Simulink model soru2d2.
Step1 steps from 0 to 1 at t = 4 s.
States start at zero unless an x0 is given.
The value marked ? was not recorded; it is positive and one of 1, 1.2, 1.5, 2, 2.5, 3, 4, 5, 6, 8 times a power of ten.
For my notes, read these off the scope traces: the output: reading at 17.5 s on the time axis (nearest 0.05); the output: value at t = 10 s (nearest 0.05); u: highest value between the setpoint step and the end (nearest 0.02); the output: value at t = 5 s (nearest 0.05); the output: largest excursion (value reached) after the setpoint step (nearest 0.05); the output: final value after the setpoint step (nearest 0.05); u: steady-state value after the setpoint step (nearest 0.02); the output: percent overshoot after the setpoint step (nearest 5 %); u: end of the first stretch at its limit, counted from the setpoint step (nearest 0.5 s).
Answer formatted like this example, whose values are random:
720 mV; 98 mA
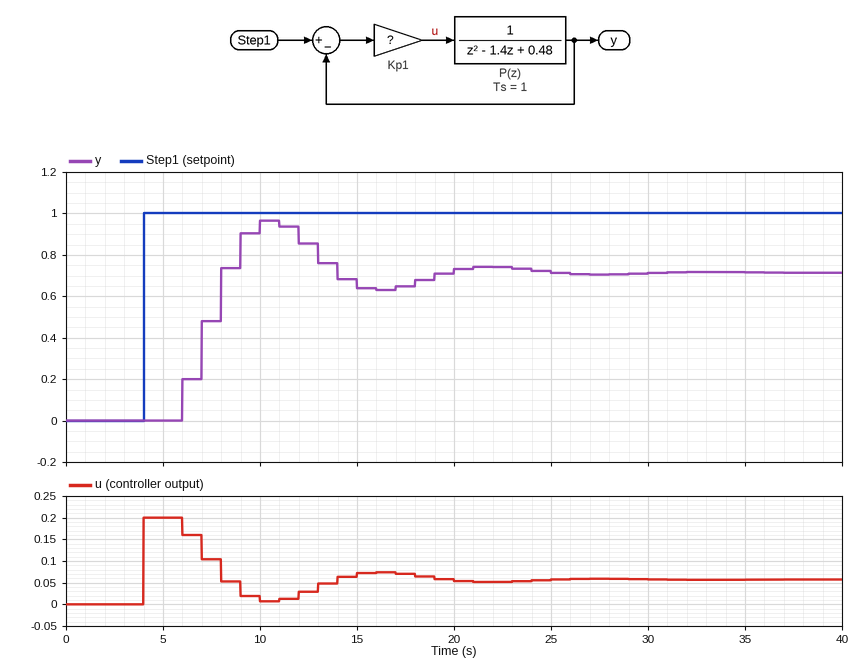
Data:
0.65; 0.95; 0.20; 0.00; 0.95; 0.70; 0.06; 35 %; 2.0 s
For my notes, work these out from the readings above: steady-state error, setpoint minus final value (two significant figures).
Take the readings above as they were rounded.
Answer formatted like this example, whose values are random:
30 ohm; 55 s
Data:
0.30
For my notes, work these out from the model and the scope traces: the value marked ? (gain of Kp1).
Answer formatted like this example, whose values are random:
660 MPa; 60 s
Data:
0.2
